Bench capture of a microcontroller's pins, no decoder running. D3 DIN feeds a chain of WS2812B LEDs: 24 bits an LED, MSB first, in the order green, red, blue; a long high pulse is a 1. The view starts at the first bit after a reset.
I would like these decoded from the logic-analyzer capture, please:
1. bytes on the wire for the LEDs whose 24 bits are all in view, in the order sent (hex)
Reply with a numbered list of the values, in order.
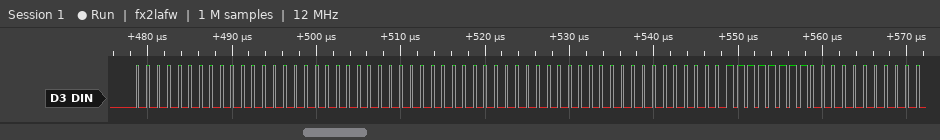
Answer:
1. 00 00 00 00 00 00 00 FF 00
